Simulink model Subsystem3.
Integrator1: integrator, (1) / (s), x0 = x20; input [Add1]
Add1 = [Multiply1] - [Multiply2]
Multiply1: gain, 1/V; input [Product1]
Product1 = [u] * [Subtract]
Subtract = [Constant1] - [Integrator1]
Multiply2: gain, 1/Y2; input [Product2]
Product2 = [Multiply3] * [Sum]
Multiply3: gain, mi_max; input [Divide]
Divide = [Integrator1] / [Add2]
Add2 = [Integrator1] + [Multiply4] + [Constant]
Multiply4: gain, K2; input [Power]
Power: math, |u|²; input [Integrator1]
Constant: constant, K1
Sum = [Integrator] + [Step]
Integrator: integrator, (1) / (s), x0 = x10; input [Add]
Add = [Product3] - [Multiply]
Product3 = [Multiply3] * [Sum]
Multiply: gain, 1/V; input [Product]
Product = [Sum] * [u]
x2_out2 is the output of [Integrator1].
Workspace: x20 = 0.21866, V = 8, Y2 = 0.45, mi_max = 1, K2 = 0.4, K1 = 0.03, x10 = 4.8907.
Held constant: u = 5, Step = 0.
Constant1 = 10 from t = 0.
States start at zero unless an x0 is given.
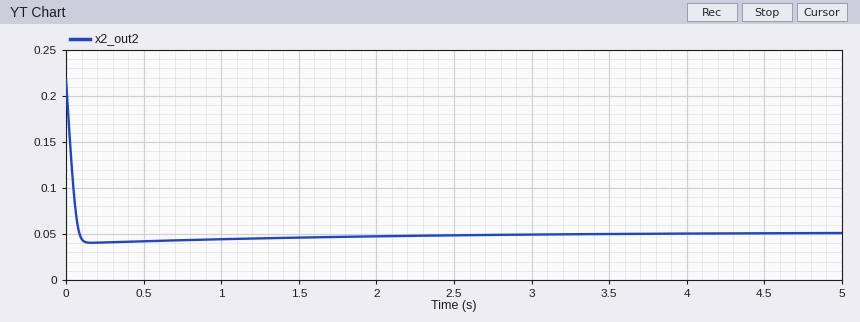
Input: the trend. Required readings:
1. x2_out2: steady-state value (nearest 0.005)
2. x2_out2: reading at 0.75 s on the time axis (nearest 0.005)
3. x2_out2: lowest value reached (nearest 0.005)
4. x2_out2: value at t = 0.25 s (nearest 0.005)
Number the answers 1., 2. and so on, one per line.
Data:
1. 0.050
2. 0.045
3. 0.040
4. 0.040
